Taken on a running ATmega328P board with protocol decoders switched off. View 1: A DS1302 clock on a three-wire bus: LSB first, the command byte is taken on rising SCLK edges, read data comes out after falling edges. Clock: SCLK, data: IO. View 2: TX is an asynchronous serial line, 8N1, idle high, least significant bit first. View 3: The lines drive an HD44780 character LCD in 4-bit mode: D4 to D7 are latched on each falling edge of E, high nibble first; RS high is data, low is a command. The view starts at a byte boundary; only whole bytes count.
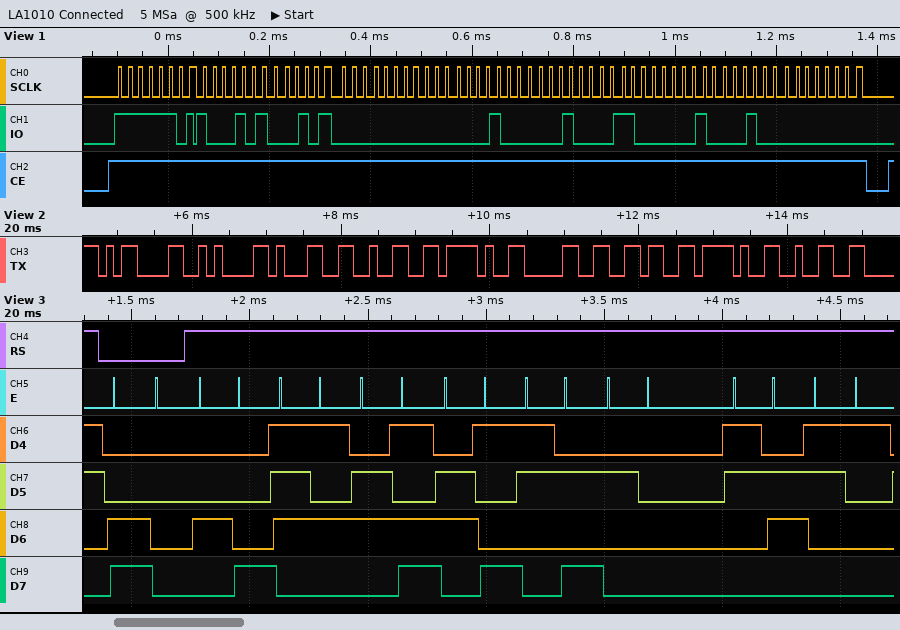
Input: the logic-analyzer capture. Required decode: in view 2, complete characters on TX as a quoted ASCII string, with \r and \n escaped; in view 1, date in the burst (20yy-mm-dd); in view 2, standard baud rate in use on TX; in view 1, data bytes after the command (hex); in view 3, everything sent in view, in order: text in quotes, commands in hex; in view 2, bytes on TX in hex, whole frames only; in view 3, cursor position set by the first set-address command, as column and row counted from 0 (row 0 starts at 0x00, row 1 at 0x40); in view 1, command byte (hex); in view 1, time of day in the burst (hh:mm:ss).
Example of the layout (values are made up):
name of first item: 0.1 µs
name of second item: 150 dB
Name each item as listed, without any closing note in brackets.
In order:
in view 2, complete characters on TX as a quoted ASCII string, with \r and \n escaped: "\r\n12/06/2"
in view 1, date in the burst: 2021-08-10
in view 2, standard baud rate in use on TX: 9600 baud
in view 1, data bytes after the command: 51 14 00 10 08 03 21 00
in view 3, everything sent in view, in order: text in quotes, commands in hex: 0xC0 "Humi: 61"
in view 2, bytes on TX in hex, whole frames only: 0D 0A 31 32 2F 30 36 2F 32
in view 3, cursor position set by the first set-address command, as column and row counted from 0: column 0, row 1
in view 1, command byte: 0xBF
in view 1, time of day in the burst: 00:14:51
